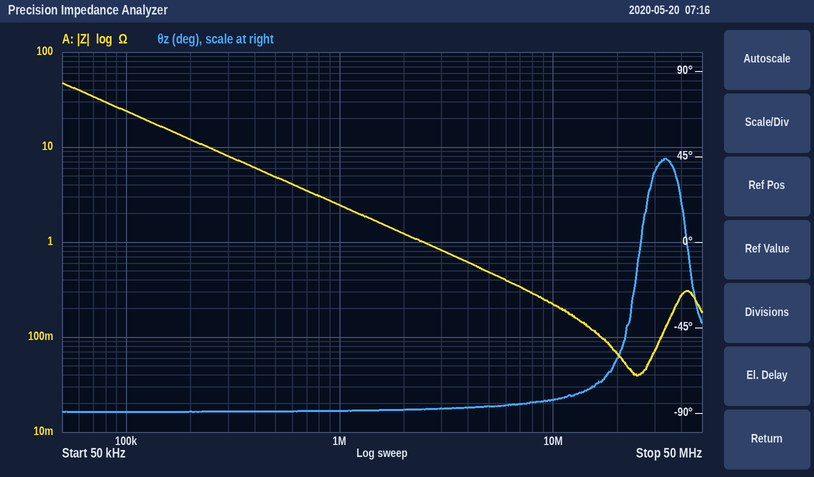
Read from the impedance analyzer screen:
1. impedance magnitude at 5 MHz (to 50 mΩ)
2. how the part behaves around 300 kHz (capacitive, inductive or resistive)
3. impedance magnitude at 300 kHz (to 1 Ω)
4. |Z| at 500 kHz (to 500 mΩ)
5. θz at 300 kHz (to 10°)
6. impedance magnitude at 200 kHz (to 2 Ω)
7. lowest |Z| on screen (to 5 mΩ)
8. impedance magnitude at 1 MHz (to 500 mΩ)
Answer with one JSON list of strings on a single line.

["500 mΩ", "capacitive", "8 Ω", "5.0 Ω", "-90°", "12 Ω", "40 mΩ", "2.5 Ω"]
